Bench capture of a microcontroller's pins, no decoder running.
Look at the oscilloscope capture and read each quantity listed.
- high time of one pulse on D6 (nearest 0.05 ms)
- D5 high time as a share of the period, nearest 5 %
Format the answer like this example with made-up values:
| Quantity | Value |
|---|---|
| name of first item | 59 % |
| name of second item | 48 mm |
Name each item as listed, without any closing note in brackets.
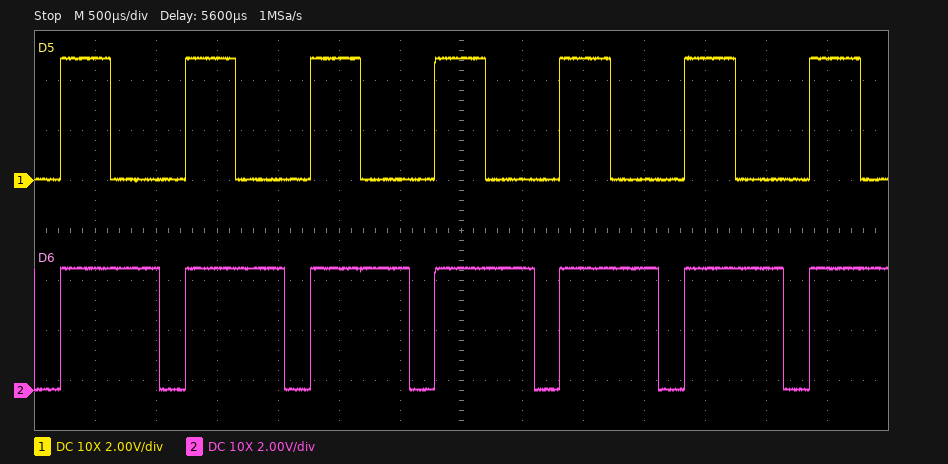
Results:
| Quantity | Value |
|---|---|
| high time of one pulse on D6 | 0.80 ms |
| D5 high time as a share of the period, nearest 5 % | 40 % |
